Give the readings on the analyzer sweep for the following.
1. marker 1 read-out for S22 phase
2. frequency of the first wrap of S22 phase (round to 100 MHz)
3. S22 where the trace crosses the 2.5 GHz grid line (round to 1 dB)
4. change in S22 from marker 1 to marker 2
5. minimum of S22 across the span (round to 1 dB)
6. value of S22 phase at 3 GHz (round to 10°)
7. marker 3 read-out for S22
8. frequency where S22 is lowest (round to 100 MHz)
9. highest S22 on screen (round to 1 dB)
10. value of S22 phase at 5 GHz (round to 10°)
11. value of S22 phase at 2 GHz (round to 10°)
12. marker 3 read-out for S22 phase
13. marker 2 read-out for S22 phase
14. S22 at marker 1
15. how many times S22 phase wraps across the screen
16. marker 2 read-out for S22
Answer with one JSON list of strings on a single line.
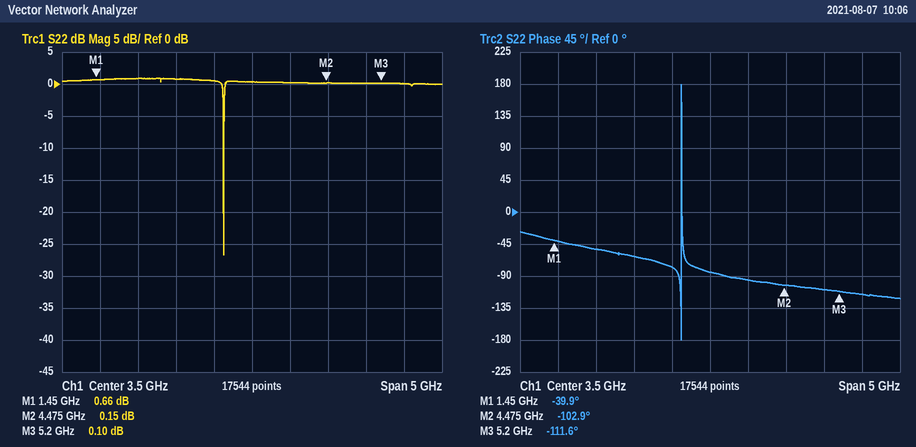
["-39.9°", "3.1 GHz", "1 dB", "-0.51 dB", "-27 dB", "-80°", "0.10 dB", "3.1 GHz", "1 dB", "-110°", "-50°", "-111.6°", "-102.9°", "0.66 dB", "1", "0.15 dB"]
